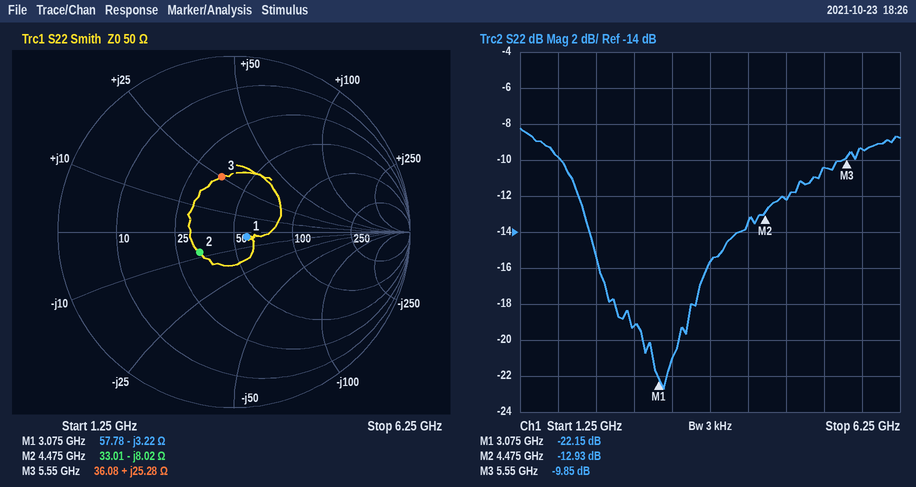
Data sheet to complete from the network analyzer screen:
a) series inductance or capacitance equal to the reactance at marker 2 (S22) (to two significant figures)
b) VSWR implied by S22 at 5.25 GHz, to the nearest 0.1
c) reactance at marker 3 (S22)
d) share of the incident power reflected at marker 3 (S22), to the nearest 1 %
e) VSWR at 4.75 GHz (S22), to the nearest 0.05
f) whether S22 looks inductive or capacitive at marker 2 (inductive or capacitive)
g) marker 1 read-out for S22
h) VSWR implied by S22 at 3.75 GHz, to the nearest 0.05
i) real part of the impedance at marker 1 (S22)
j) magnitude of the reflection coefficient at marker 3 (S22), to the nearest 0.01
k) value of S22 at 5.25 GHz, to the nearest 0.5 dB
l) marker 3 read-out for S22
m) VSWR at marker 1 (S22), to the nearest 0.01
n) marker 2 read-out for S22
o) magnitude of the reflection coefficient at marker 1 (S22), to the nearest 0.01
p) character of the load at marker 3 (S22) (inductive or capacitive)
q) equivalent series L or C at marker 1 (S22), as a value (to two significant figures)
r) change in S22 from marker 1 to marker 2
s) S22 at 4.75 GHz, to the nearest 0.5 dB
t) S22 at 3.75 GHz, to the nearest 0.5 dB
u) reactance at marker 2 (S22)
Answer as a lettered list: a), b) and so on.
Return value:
a) 4.4 pF
b) 1.9
c) +25.28 Ω
d) 10 %
e) 1.65
f) capacitive
g) -22.15 dB
h) 1.40
i) 57.78 Ω
j) 0.32
k) -10.5 dB
l) -9.85 dB
m) 1.17
n) -12.93 dB
o) 0.08
p) inductive
q) 16 pF
r) 9.22 dB
s) -12.0 dB
t) -15.5 dB
u) -8.02 Ω
